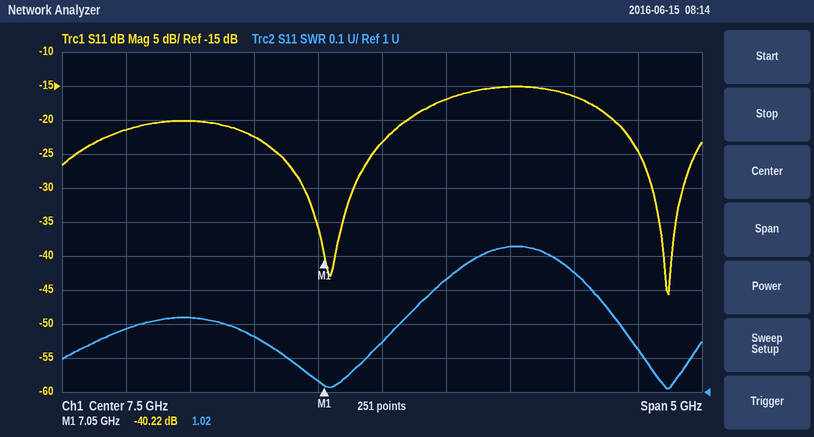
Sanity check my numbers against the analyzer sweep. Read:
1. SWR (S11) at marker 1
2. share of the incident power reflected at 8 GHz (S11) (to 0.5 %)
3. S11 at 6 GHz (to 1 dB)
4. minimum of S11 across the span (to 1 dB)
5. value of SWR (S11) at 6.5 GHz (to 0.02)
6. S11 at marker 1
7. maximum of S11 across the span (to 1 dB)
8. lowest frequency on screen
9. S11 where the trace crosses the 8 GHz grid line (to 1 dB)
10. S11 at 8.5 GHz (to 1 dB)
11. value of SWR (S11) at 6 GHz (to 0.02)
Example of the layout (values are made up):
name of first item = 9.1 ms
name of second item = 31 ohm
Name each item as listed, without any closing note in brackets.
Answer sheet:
SWR (S11) at marker 1 = 1.02
share of the incident power reflected at 8 GHz (S11) = 2.0 %
S11 at 6 GHz = -20 dB
minimum of S11 across the span = -46 dB
value of SWR (S11) at 6.5 GHz = 1.16
S11 at marker 1 = -40.22 dB
maximum of S11 across the span = -15 dB
lowest frequency on screen = 5 GHz
S11 where the trace crosses the 8 GHz grid line = -17 dB
S11 at 8.5 GHz = -15 dB
value of SWR (S11) at 6 GHz = 1.22
